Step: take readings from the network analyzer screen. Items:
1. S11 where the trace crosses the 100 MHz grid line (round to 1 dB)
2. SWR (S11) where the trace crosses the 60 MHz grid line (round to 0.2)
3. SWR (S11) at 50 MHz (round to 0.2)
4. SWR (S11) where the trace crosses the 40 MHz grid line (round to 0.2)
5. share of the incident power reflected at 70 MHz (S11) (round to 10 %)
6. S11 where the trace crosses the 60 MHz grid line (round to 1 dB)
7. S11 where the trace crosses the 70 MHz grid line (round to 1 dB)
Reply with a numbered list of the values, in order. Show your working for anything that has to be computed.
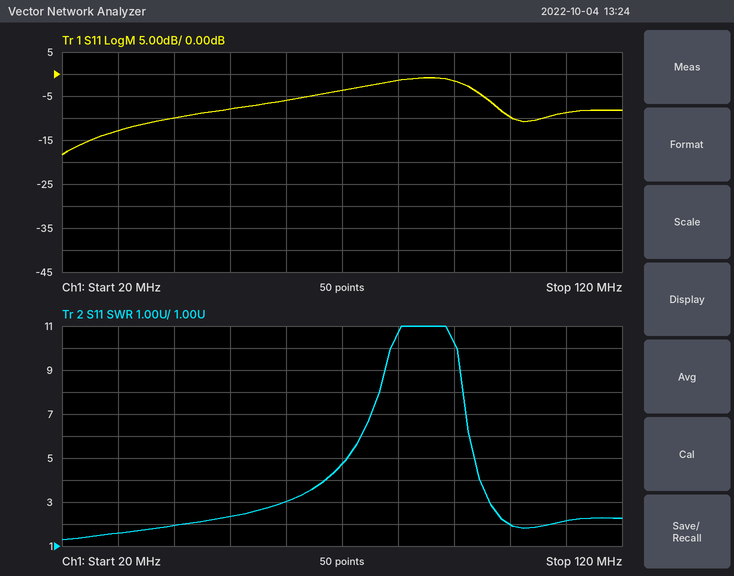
1. -10 dB
2. 3.0
3. 2.4
4. 2.0
5. 10^(-4/10) ≈ 40 %
6. -6 dB
7. -4 dB
